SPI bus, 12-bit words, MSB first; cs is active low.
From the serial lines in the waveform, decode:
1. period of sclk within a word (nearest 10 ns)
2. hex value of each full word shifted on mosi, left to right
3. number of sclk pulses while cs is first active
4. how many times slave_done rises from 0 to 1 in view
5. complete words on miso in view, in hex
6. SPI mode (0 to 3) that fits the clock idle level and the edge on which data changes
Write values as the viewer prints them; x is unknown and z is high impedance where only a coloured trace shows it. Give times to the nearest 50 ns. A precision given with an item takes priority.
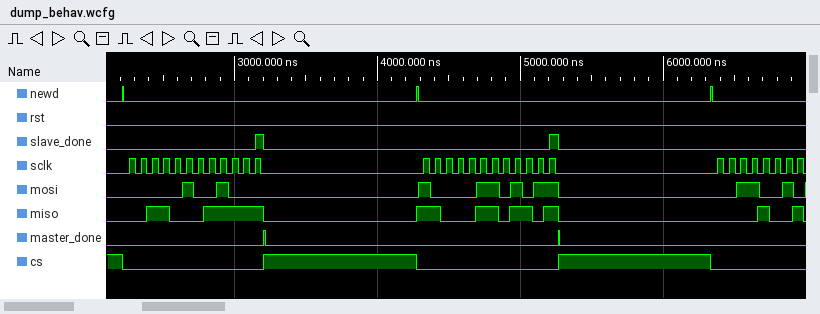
80 ns
048, 86B
12
2
31F, C6D
0
